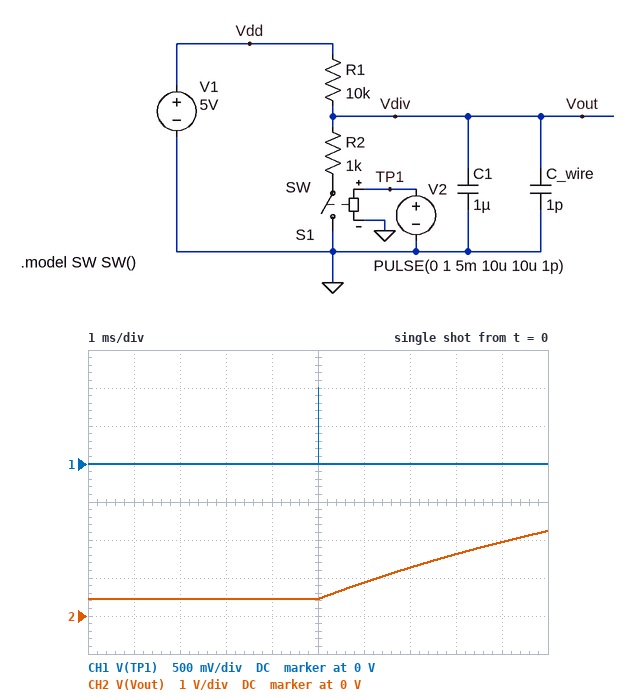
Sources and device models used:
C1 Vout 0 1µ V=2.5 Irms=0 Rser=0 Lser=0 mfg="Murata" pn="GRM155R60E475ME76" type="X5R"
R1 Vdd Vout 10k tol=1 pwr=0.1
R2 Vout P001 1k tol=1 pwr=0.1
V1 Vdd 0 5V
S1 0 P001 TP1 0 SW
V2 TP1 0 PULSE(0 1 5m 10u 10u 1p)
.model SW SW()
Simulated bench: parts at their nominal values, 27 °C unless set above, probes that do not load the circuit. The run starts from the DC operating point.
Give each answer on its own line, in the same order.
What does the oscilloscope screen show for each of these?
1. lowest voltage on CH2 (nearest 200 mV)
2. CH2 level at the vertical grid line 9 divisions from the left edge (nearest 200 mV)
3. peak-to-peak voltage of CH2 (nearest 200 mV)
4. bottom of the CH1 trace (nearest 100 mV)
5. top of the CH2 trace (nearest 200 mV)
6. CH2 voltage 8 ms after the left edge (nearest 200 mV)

400 mV
2.0 V
1.8 V
0 V
2.2 V
1.6 V
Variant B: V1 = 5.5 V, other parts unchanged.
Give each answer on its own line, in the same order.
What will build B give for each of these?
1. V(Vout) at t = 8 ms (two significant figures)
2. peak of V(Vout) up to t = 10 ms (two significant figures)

1.8 V
2.5 V
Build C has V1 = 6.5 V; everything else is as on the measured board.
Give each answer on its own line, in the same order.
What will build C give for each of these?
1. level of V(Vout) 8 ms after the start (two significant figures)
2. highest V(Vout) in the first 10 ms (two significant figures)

2.1 V
2.9 V
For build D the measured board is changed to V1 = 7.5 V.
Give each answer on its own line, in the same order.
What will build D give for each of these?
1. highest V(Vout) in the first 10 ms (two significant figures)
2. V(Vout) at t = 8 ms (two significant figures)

3.4 V
2.4 V
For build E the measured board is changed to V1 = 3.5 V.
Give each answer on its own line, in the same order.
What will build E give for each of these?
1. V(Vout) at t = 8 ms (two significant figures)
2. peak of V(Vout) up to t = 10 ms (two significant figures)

1.1 V
1.6 V
